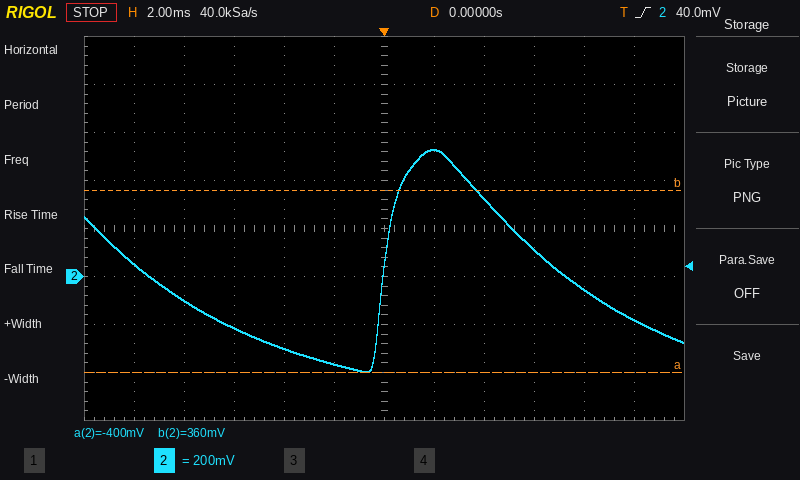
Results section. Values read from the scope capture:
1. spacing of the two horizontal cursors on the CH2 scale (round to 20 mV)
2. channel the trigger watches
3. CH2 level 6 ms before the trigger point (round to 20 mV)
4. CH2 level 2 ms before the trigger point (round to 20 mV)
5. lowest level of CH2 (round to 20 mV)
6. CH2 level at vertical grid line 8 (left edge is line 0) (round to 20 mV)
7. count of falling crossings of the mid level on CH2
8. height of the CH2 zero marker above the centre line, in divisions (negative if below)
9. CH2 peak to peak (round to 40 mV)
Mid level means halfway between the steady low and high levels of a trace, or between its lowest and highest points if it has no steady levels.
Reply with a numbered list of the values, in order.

1. 760 mV
2. CH2
3. -220 mV
4. -360 mV
5. -400 mV
6. 320 mV
7. 2
8. -1.0 div
9. 920 mV
